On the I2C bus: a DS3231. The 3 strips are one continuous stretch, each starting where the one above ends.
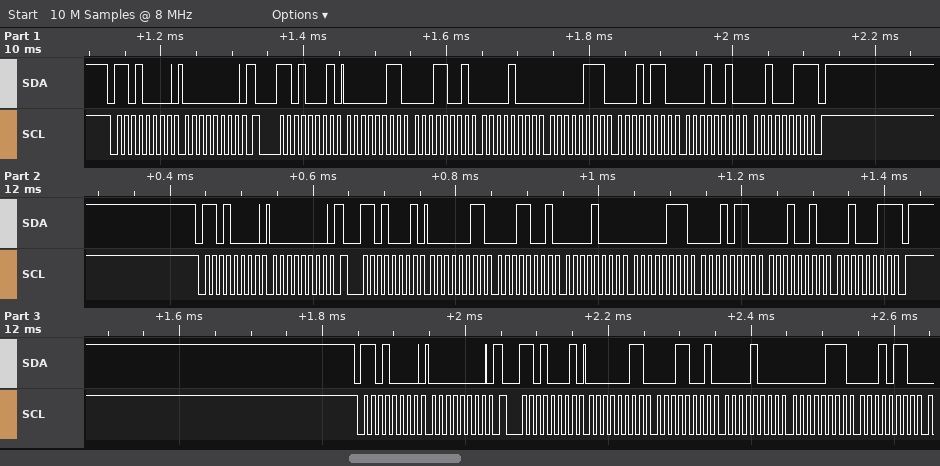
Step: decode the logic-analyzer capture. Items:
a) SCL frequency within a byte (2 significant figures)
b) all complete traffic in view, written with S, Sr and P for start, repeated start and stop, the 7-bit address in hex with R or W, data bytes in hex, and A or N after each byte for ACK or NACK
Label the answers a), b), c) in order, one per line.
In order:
a) 100 kHz
b) S 68W A 00 A Sr 68R A 03 A 19 A 08 A 07 A 16 A 12 A 23 N P S 68W A 00 A Sr 68R A 03 A 19 A 08 A 07 A 16 A 12 A 23 N P S 68W A 00 A Sr 68R A 03 A 19 A 08 A 07 A 16 A
